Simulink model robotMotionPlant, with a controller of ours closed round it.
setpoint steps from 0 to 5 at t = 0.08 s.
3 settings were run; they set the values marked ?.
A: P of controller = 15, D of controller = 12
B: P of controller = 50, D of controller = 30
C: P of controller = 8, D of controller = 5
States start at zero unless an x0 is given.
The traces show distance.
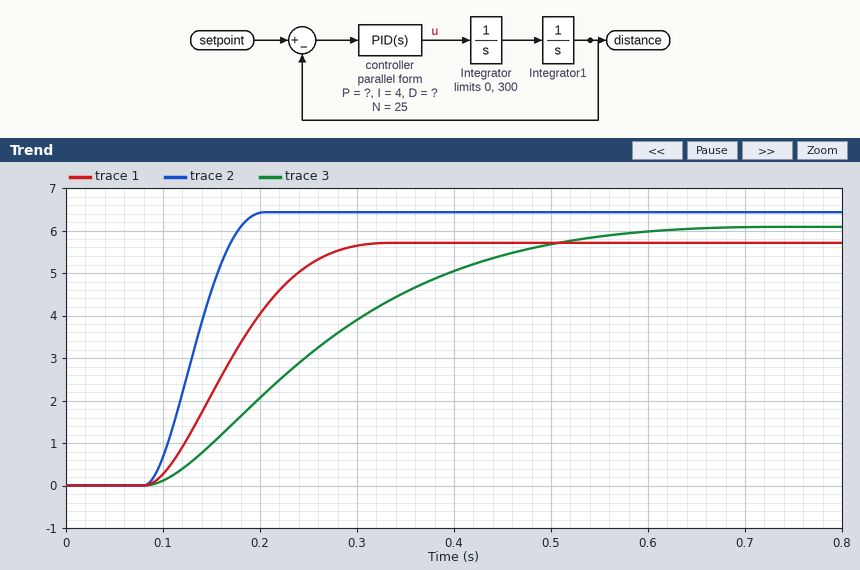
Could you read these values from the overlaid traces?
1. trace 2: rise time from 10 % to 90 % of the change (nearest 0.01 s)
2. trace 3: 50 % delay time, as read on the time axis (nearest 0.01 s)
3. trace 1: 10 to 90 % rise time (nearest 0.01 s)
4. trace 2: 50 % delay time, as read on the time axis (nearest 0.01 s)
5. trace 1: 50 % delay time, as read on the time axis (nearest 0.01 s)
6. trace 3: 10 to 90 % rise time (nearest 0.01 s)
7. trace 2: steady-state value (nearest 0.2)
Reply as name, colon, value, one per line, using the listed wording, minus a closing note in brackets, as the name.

trace 2: rise time from 10 % to 90 % of the change: 0.07 s
trace 3: 50 % delay time, as read on the time axis: 0.25 s
trace 1: 10 to 90 % rise time: 0.14 s
trace 2: 50 % delay time, as read on the time axis: 0.13 s
trace 1: 50 % delay time, as read on the time axis: 0.17 s
trace 3: 10 to 90 % rise time: 0.33 s
trace 2: steady-state value: 6.4
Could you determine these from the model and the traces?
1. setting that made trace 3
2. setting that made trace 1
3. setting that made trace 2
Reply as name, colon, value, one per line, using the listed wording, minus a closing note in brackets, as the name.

setting that made trace 3: C
setting that made trace 1: A
setting that made trace 2: B
